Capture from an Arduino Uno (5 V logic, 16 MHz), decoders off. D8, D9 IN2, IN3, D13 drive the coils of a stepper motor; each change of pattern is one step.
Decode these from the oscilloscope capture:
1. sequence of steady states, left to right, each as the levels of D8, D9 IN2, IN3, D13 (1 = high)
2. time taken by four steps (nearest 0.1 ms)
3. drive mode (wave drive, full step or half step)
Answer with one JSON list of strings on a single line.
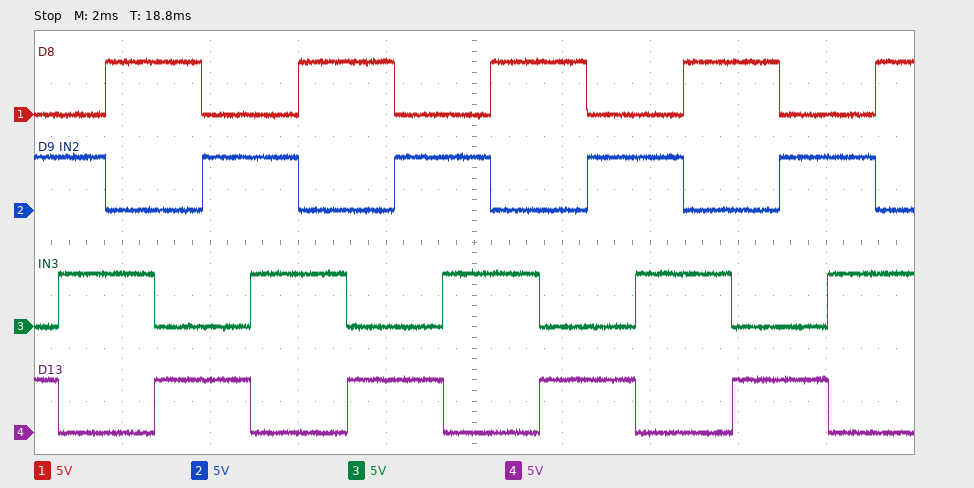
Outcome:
["0101 0110 1010 1001 0101 0110 1010 1001 0101 0110 1010 1001 0101 0110 1010 1001 0101 0110 1010", "4.4 ms", "full step"]
